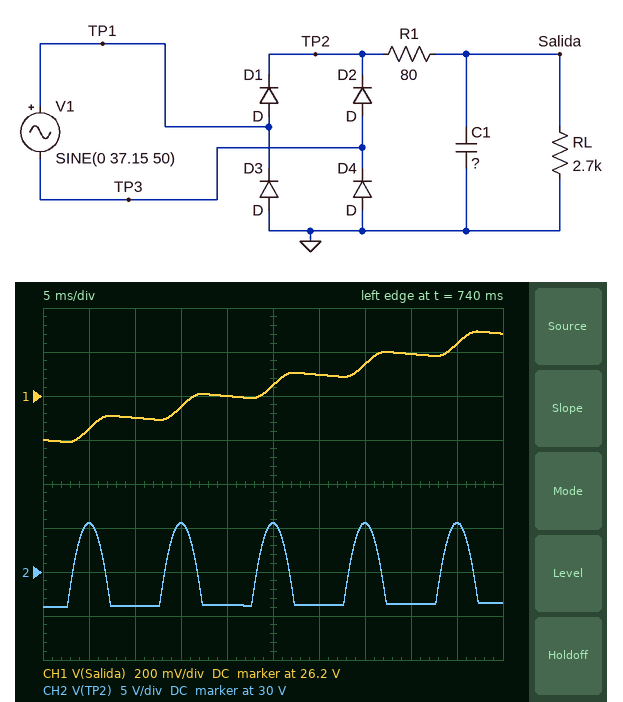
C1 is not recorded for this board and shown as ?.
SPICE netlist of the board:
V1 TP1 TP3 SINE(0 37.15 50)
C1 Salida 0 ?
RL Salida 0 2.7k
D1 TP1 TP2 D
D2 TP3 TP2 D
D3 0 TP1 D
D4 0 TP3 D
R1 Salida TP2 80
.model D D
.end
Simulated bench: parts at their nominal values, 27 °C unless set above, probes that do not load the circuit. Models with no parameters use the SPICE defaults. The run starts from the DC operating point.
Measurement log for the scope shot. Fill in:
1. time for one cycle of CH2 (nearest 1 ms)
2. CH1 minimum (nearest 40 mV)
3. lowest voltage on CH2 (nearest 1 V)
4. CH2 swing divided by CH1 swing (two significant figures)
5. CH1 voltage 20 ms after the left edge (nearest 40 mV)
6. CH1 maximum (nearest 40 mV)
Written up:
10 ms
26.00 V
26 V
19
26.20 V
26.48 V
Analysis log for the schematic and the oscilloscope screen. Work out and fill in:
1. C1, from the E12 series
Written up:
2.7 mF
